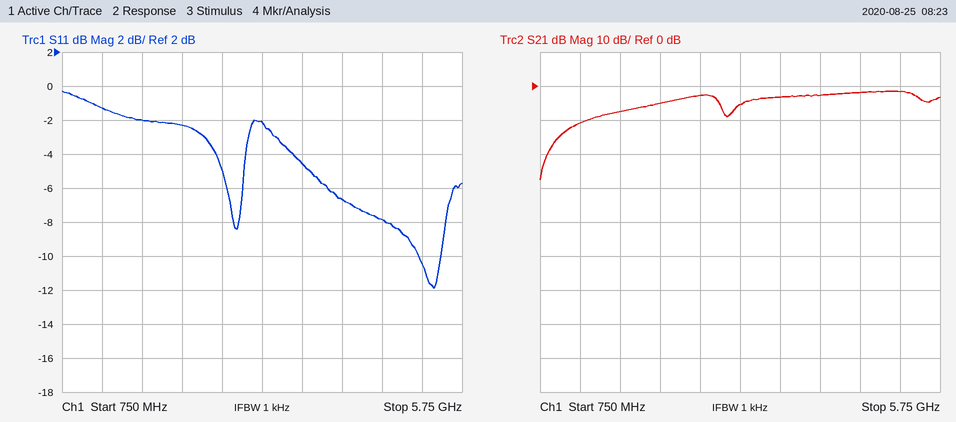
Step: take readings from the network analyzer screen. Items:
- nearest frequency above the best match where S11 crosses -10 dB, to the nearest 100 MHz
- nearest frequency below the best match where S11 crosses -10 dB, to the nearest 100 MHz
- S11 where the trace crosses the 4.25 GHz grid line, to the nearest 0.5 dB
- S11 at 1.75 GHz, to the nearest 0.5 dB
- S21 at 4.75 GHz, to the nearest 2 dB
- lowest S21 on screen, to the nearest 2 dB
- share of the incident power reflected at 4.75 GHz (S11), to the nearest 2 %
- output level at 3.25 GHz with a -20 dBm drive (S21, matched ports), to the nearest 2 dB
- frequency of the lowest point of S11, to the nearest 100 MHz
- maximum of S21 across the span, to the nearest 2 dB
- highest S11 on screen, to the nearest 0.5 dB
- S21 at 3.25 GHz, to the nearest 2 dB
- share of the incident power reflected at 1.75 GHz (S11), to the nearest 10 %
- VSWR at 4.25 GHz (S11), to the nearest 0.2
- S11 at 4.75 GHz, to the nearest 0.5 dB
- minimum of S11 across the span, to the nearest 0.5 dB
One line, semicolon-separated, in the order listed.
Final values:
5.5 GHz; 5.2 GHz; -6.5 dB; -2.0 dB; -2 dB; -28 dB; 16 %; -26 dBm; 5.4 GHz; -2 dB; -0.5 dB; -6 dB; 60 %; 2.8; -8.0 dB; -12.0 dB
